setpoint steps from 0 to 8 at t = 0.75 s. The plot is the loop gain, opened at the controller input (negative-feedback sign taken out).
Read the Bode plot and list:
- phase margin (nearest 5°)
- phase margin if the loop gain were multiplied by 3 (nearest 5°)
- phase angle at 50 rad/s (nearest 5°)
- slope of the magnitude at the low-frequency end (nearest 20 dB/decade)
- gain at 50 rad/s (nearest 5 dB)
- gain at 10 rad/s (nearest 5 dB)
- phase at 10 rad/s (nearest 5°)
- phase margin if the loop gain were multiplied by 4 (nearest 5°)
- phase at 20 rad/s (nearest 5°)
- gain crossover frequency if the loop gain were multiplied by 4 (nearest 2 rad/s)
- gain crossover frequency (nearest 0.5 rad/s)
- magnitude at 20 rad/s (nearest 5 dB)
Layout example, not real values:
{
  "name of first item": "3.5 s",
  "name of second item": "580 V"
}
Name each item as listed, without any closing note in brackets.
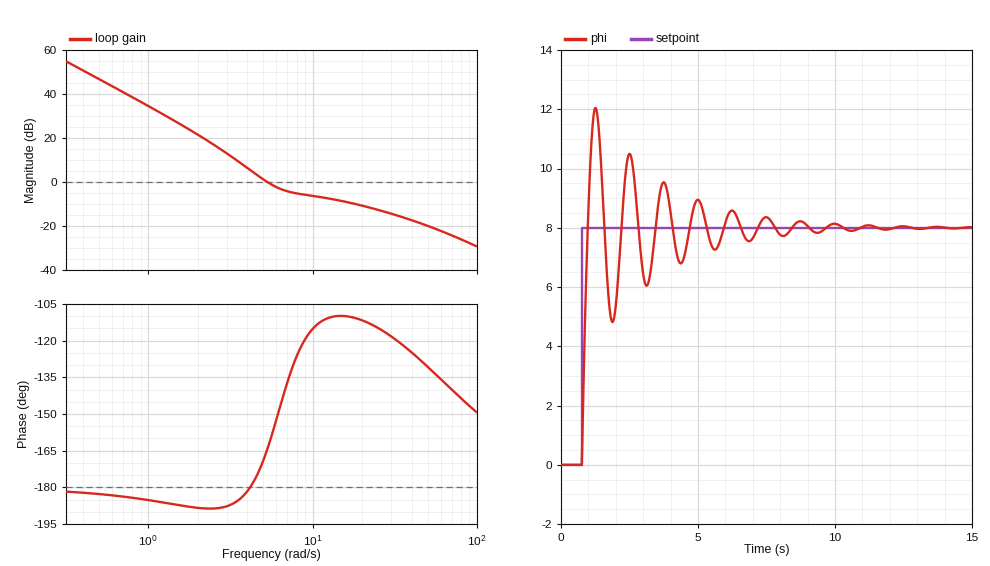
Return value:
{
  "phase margin": "15°",
  "phase margin if the loop gain were multiplied by 3": "70°",
  "phase angle at 50 rad/s": "-130°",
  "slope of the magnitude at the low-frequency end": "-40 dB/decade",
  "gain at 50 rad/s": "-20 dB",
  "gain at 10 rad/s": "-5 dB",
  "phase at 10 rad/s": "-115°",
  "phase margin if the loop gain were multiplied by 4": "65°",
  "phase at 20 rad/s": "-110°",
  "gain crossover frequency if the loop gain were multiplied by 4": "24 rad/s",
  "gain crossover frequency": "5.5 rad/s",
  "magnitude at 20 rad/s": "-10 dB"
}
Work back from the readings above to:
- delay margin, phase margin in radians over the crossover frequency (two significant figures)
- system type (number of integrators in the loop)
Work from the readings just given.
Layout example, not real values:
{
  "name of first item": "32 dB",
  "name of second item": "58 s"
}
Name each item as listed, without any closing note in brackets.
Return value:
{
  "delay margin, phase margin in radians over the crossover frequency": "0.048 s",
  "system type": "2"
}
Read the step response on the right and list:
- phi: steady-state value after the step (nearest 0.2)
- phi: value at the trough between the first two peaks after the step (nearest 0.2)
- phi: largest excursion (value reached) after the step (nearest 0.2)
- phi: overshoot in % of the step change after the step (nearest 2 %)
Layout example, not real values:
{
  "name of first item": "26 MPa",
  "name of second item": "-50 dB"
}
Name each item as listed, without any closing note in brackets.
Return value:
{
  "phi: steady-state value after the step": "8.0",
  "phi: value at the trough between the first two peaks after the step": "4.8",
  "phi: largest excursion (value reached) after the step": "12.0",
  "phi: overshoot in % of the step change after the step": "50 %"
}
